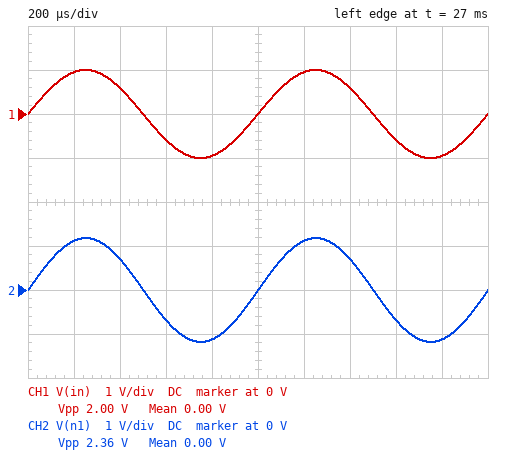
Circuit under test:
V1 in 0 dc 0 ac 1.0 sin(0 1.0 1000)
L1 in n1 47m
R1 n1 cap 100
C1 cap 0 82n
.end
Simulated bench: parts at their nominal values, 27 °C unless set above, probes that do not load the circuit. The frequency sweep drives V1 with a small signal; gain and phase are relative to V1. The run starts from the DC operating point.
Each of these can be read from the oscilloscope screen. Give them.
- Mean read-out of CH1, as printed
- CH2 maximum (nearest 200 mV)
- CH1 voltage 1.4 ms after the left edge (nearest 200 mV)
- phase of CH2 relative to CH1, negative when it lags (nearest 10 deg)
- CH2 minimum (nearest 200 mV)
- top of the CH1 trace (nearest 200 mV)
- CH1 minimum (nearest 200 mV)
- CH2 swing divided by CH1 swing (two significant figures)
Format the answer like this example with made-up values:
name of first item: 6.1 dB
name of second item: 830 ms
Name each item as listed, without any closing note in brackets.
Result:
Mean read-out of CH1, as printed: 0.00 V
CH2 maximum: 1.2 V
CH1 voltage 1.4 ms after the left edge: 600 mV
phase of CH2 relative to CH1, negative when it lags: 0 deg
CH2 minimum: -1.2 V
top of the CH1 trace: 1.0 V
CH1 minimum: -1.0 V
CH2 swing divided by CH1 swing: 1.2
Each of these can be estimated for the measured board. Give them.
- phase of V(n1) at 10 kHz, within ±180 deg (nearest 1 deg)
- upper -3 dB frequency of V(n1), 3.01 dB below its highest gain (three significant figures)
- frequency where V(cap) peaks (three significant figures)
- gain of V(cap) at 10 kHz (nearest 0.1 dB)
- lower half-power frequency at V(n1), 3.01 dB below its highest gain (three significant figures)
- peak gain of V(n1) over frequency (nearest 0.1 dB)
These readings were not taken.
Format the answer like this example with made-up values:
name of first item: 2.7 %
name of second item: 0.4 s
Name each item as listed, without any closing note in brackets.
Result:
phase of V(n1) at 10 kHz, within ±180 deg: -151 deg
upper -3 dB frequency of V(n1), 3.01 dB below its highest gain: 2.72 kHz
frequency where V(cap) peaks: 2.55 kHz
gain of V(cap) at 10 kHz: -23.1 dB
lower half-power frequency at V(n1), 3.01 dB below its highest gain: 2.38 kHz
peak gain of V(n1) over frequency: 17.7 dB
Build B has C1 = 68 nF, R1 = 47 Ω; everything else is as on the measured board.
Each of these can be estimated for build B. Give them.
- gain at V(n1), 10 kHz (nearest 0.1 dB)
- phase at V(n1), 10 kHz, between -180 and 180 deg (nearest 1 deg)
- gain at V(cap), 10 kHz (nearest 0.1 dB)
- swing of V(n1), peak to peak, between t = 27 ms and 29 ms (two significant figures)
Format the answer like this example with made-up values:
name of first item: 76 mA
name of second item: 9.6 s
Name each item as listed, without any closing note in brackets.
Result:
gain at V(n1), 10 kHz: -21.1 dB
phase at V(n1), 10 kHz, between -180 and 180 deg: -168 deg
gain at V(cap), 10 kHz: -21.3 dB
swing of V(n1), peak to peak, between t = 27 ms and 29 ms: 2.3 V
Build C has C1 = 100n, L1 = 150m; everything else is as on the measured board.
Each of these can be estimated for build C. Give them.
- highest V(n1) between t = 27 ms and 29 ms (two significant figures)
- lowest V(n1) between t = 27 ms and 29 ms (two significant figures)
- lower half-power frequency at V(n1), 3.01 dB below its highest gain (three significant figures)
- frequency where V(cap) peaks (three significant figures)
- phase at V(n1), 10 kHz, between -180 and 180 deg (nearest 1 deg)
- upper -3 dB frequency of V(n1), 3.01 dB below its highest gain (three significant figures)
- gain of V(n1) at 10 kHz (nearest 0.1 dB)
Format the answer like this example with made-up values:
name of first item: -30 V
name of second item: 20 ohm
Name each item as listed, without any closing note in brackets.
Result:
highest V(n1) between t = 27 ms and 29 ms: 2.4 V
lowest V(n1) between t = 27 ms and 29 ms: -2.4 V
lower half-power frequency at V(n1), 3.01 dB below its highest gain: 1.24 kHz
frequency where V(cap) peaks: 1.30 kHz
phase at V(n1), 10 kHz, between -180 and 180 deg: -147 deg
upper -3 dB frequency of V(n1), 3.01 dB below its highest gain: 1.35 kHz
gain of V(n1) at 10 kHz: -33.9 dB
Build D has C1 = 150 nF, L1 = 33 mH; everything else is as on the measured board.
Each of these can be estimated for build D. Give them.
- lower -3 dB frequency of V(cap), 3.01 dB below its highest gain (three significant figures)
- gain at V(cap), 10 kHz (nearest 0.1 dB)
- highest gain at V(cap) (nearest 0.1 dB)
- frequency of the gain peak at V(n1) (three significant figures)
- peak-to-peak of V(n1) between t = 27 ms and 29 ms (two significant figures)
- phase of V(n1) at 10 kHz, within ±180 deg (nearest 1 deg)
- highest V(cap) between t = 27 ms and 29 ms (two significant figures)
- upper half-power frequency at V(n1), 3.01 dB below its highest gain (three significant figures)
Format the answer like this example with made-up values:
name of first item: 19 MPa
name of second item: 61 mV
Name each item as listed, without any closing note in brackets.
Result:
lower -3 dB frequency of V(cap), 3.01 dB below its highest gain: 1.98 kHz
gain at V(cap), 10 kHz: -25.4 dB
highest gain at V(cap): 13.5 dB
frequency of the gain peak at V(n1): 2.24 kHz
peak-to-peak of V(n1) between t = 27 ms and 29 ms: 2.5 V
phase of V(n1) at 10 kHz, within ±180 deg: -134 deg
highest V(cap) between t = 27 ms and 29 ms: 1.2 V
upper half-power frequency at V(n1), 3.01 dB below its highest gain: 2.47 kHz
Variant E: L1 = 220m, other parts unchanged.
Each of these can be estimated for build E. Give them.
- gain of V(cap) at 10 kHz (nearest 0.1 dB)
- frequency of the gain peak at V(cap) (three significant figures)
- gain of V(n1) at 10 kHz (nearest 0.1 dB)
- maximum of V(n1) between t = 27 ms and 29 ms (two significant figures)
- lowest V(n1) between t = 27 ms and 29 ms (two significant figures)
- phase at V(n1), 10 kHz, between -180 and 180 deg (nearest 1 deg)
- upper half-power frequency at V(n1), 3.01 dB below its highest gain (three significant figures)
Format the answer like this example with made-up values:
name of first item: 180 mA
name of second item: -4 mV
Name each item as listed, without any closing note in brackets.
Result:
gain of V(cap) at 10 kHz: -36.9 dB
frequency of the gain peak at V(cap): 1.18 kHz
gain of V(n1) at 10 kHz: -35.9 dB
maximum of V(n1) between t = 27 ms and 29 ms: 3.4 V
lowest V(n1) between t = 27 ms and 29 ms: -3.4 V
phase at V(n1), 10 kHz, between -180 and 180 deg: -152 deg
upper half-power frequency at V(n1), 3.01 dB below its highest gain: 1.22 kHz
